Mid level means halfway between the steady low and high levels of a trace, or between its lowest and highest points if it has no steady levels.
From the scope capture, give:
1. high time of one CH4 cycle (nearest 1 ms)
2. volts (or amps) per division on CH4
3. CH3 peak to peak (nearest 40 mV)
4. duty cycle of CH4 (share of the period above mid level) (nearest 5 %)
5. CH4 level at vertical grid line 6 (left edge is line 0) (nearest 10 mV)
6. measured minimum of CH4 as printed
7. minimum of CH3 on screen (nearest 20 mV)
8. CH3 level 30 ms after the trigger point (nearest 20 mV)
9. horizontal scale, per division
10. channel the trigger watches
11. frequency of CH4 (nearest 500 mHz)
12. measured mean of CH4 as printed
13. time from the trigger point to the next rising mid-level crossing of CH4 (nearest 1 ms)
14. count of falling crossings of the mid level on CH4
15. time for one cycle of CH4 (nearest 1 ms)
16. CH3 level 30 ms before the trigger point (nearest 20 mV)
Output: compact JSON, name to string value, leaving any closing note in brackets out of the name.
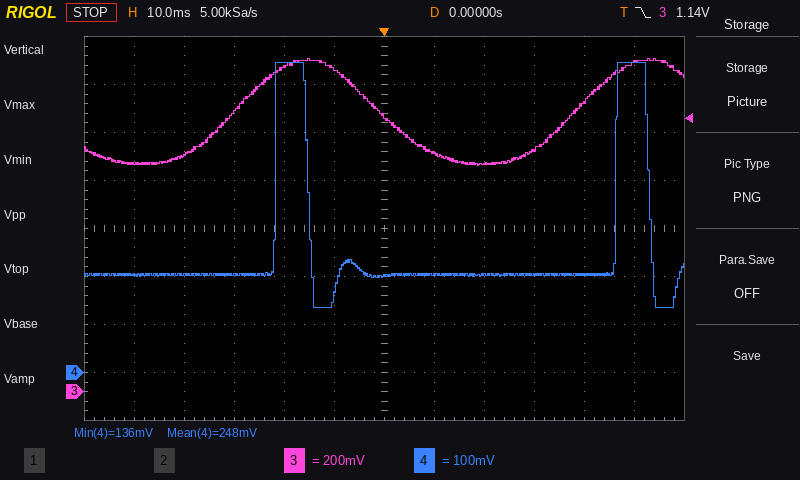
{"high time of one CH4 cycle": "7 ms", "volts (or amps) per division on CH4": "100 mV", "CH3 peak to peak": "440 mV", "duty cycle of CH4 (share of the period above mid level)": "10 %", "CH4 level at vertical grid line 6 (left edge is line 0)": "200 mV", "measured minimum of CH4 as printed": "136 mV", "minimum of CH3 on screen": "940 mV", "CH3 level 30 ms after the trigger point": "1.00 V", "horizontal scale, per division": "10 ms", "channel the trigger watches": "CH3", "frequency of CH4": "14.5 Hz", "measured mean of CH4 as printed": "248 mV", "time from the trigger point to the next rising mid-level crossing of CH4": "46 ms", "count of falling crossings of the mid level on CH4": "2", "time for one cycle of CH4": "68 ms", "CH3 level 30 ms before the trigger point": "1.16 V"}
